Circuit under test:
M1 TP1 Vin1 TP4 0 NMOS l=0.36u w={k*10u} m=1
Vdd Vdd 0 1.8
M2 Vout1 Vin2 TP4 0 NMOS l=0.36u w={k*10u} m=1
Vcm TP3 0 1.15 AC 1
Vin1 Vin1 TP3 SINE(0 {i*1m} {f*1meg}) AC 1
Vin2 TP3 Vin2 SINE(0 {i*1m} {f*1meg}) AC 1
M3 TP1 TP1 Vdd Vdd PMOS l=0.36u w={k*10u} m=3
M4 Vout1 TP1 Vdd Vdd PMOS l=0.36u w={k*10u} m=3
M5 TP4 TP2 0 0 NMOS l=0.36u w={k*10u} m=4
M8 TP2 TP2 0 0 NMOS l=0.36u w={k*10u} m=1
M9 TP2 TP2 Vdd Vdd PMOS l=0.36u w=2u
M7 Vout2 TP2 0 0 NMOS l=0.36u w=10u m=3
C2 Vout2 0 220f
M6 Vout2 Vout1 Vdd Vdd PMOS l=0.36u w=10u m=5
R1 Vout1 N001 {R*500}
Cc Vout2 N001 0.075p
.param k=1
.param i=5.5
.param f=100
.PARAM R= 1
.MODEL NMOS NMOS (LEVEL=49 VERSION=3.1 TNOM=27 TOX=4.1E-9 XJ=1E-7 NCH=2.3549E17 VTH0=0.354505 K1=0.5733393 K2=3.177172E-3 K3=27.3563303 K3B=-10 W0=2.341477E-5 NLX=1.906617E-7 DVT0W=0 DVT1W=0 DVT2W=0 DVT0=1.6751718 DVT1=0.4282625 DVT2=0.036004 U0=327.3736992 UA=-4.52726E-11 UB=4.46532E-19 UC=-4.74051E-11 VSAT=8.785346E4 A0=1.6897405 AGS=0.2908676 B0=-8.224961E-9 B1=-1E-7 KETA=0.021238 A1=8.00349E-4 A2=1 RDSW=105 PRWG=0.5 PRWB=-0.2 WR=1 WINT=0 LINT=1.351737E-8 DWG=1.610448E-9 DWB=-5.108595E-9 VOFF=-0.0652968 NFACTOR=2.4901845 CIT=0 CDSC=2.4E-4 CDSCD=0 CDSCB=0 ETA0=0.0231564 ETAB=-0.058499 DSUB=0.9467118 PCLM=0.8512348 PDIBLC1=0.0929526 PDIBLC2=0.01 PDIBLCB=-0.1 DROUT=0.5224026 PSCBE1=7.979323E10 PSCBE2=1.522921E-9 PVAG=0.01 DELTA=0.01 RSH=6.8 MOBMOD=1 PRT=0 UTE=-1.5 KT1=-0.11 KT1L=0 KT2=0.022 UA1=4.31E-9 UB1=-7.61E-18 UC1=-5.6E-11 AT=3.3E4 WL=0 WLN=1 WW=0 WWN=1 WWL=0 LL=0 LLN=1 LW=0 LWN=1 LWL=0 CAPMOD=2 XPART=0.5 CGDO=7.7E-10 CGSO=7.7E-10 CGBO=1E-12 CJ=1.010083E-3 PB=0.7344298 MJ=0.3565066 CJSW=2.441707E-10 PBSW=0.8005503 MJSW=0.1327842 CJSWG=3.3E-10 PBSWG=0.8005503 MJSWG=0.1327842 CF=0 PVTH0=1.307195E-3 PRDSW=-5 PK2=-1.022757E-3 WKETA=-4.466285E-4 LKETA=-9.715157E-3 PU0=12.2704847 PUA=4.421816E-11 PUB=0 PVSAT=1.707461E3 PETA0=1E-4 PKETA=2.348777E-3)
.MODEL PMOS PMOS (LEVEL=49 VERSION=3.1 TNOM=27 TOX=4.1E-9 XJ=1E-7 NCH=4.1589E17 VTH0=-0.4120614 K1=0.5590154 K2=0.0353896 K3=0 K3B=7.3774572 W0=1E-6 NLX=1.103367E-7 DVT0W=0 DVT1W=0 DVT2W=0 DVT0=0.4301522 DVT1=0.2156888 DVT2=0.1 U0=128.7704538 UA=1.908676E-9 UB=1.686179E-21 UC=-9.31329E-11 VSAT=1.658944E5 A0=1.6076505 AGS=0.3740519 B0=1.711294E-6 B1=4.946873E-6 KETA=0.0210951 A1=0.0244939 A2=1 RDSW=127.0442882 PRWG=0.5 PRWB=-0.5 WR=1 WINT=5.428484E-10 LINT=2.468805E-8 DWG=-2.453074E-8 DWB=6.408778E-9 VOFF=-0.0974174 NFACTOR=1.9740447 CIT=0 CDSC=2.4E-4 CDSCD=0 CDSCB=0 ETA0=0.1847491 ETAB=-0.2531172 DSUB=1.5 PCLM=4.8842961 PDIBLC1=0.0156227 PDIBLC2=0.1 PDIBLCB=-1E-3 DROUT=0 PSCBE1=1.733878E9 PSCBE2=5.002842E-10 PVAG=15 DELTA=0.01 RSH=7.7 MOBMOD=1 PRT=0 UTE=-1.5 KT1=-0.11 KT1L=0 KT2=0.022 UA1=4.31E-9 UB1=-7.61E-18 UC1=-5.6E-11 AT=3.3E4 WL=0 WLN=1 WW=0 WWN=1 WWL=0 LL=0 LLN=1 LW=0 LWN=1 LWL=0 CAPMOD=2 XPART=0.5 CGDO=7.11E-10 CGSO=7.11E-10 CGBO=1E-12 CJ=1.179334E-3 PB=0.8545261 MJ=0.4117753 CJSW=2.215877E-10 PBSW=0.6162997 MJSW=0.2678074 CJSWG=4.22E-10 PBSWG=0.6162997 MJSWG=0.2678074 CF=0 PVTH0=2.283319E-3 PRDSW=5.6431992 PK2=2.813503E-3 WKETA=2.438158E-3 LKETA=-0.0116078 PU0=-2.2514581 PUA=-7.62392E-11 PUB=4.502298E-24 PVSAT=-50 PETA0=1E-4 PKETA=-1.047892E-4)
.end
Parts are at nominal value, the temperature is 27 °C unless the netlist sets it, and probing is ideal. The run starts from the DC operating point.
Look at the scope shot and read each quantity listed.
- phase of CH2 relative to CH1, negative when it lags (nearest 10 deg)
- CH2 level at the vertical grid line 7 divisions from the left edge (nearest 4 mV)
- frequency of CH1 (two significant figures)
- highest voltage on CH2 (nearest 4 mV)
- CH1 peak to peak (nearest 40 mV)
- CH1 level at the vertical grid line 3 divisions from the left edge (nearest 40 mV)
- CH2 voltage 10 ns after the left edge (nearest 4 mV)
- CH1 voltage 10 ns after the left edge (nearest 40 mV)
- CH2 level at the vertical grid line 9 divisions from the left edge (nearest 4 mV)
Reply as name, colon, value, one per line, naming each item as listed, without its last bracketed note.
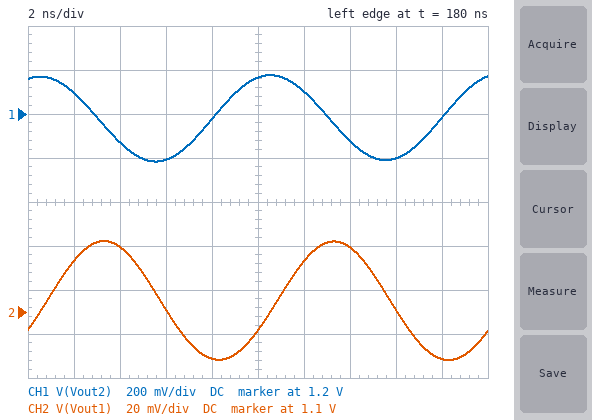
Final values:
phase of CH2 relative to CH1, negative when it lags: -100 deg
CH2 level at the vertical grid line 7 divisions from the left edge: 1.128 V
frequency of CH1: 100 MHz
highest voltage on CH2: 1.132 V
CH1 peak to peak: 400 mV
CH1 level at the vertical grid line 3 divisions from the left edge: 1.00 V
CH2 voltage 10 ns after the left edge: 1.092 V
CH1 voltage 10 ns after the left edge: 1.36 V
CH2 level at the vertical grid line 9 divisions from the left edge: 1.080 V
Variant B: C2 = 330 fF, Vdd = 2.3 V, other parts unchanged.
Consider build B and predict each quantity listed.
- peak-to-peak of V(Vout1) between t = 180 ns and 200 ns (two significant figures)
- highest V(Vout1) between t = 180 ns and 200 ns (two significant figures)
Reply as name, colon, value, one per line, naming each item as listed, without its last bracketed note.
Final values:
peak-to-peak of V(Vout1) between t = 180 ns and 200 ns: 62 mV
highest V(Vout1) between t = 180 ns and 200 ns: 1.5 V
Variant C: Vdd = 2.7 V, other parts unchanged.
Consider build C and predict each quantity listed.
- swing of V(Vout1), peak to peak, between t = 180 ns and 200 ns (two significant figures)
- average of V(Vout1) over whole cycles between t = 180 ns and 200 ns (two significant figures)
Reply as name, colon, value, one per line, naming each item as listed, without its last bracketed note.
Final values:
swing of V(Vout1), peak to peak, between t = 180 ns and 200 ns: 50 mV
average of V(Vout1) over whole cycles between t = 180 ns and 200 ns: 1.8 V
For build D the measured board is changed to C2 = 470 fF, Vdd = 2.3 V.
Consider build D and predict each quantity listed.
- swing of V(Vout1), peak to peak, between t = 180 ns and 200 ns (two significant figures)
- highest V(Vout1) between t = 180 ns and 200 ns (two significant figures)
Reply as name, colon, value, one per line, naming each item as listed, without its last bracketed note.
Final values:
swing of V(Vout1), peak to peak, between t = 180 ns and 200 ns: 74 mV
highest V(Vout1) between t = 180 ns and 200 ns: 1.5 V
